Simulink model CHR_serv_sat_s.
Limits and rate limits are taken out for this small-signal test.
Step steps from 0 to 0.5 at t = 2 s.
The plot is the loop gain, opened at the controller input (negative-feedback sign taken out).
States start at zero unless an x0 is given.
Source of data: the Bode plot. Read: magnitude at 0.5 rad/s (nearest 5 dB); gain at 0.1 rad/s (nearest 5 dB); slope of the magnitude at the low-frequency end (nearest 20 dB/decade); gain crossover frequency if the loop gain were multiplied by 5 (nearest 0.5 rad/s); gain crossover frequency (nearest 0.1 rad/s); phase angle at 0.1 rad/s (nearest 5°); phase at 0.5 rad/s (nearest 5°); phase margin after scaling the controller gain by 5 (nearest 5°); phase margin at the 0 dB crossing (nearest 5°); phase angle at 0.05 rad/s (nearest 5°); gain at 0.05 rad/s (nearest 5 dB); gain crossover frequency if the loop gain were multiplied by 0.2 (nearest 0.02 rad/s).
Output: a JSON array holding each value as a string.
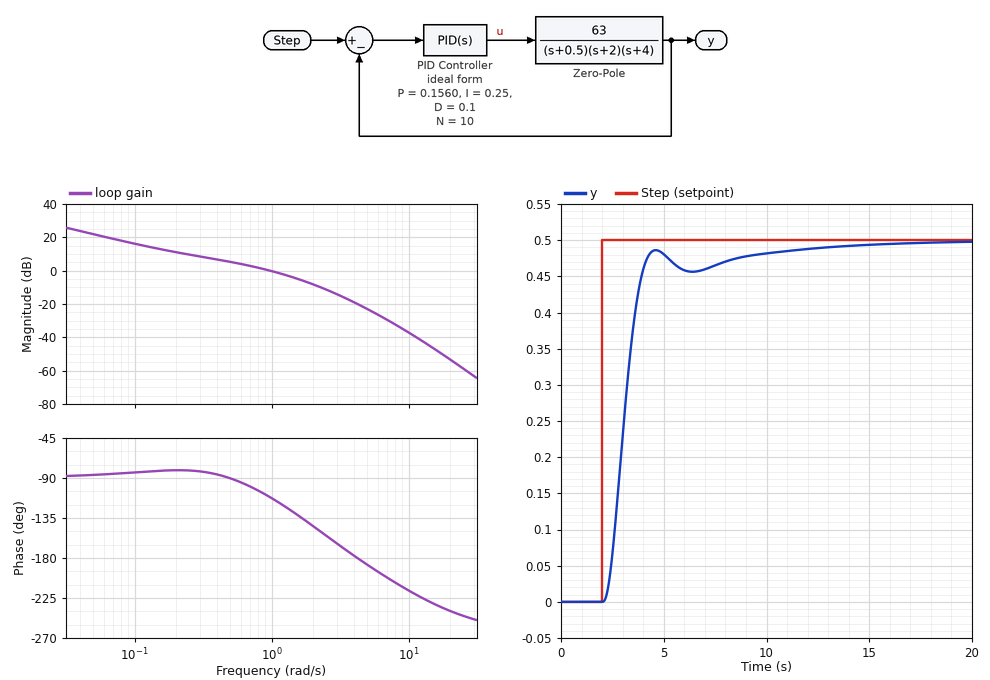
["5 dB", "15 dB", "-20 dB/decade", "3.0 rad/s", "1.0 rad/s", "-85°", "-90°", "15°", "70°", "-85°", "20 dB", "0.14 rad/s"]
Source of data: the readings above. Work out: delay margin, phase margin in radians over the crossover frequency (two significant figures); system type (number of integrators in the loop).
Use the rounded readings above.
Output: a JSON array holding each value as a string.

["1.2 s", "1"]
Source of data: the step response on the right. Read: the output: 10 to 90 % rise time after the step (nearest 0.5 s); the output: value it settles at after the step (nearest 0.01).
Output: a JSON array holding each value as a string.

["1.5 s", "0.50"]
